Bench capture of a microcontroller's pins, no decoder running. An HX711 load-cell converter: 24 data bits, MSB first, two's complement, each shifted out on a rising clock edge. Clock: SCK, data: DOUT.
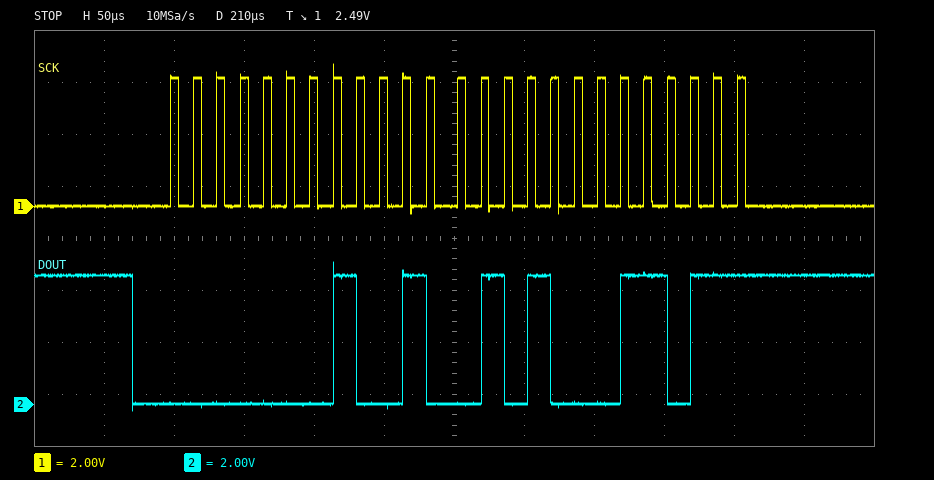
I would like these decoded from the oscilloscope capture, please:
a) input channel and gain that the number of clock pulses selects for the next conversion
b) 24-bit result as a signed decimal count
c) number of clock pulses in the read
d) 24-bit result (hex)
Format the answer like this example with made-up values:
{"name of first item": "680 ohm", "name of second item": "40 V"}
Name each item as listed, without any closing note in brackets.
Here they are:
{"input channel and gain that the number of clock pulses selects for the next conversion": "channel A, gain 128", "24-bit result as a signed decimal count": "75035", "number of clock pulses in the read": "25", "24-bit result": "0x01251B"}
